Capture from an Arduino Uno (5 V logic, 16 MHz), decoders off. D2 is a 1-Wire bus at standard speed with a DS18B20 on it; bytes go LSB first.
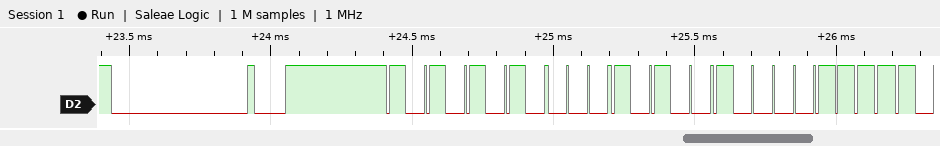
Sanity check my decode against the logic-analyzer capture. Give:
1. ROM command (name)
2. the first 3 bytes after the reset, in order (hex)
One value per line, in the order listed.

Match ROM
55 28 E1
